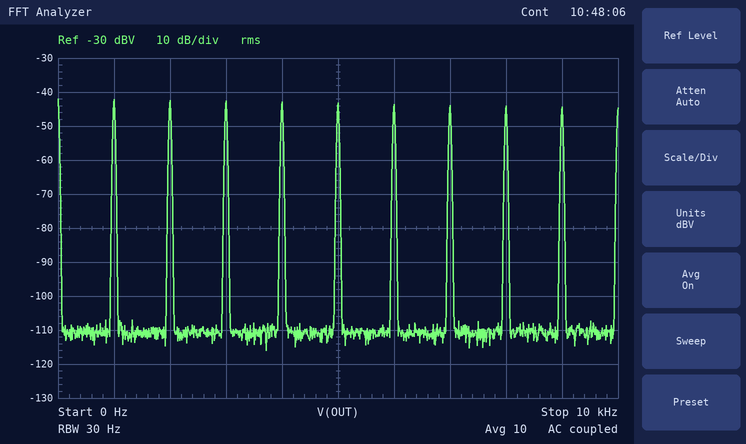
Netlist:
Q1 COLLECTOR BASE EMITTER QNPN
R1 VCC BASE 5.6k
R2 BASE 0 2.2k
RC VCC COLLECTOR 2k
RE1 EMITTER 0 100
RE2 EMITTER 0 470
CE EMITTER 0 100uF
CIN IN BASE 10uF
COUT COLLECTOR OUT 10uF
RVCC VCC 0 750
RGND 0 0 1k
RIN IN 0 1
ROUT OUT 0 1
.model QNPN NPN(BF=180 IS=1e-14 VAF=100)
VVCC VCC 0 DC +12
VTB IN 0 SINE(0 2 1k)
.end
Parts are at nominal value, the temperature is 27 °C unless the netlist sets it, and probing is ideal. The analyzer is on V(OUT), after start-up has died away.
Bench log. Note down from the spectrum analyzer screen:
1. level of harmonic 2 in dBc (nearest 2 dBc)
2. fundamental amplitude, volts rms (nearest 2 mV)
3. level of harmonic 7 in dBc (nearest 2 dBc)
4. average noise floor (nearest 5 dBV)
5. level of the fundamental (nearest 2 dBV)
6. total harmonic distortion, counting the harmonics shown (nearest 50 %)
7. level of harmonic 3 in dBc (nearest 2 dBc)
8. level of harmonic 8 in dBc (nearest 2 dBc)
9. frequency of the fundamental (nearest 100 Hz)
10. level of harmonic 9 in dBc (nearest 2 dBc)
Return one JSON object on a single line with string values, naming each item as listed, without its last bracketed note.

{"level of harmonic 2 in dBc": "0 dBc", "fundamental amplitude, volts rms": "8 mV", "level of harmonic 7 in dBc": "-2 dBc", "average noise floor": "-110 dBV", "level of the fundamental": "-42 dBV", "total harmonic distortion, counting the harmonics shown": "250 %", "level of harmonic 3 in dBc": "0 dBc", "level of harmonic 8 in dBc": "-2 dBc", "frequency of the fundamental": "1.0 kHz", "level of harmonic 9 in dBc": "-2 dBc"}
